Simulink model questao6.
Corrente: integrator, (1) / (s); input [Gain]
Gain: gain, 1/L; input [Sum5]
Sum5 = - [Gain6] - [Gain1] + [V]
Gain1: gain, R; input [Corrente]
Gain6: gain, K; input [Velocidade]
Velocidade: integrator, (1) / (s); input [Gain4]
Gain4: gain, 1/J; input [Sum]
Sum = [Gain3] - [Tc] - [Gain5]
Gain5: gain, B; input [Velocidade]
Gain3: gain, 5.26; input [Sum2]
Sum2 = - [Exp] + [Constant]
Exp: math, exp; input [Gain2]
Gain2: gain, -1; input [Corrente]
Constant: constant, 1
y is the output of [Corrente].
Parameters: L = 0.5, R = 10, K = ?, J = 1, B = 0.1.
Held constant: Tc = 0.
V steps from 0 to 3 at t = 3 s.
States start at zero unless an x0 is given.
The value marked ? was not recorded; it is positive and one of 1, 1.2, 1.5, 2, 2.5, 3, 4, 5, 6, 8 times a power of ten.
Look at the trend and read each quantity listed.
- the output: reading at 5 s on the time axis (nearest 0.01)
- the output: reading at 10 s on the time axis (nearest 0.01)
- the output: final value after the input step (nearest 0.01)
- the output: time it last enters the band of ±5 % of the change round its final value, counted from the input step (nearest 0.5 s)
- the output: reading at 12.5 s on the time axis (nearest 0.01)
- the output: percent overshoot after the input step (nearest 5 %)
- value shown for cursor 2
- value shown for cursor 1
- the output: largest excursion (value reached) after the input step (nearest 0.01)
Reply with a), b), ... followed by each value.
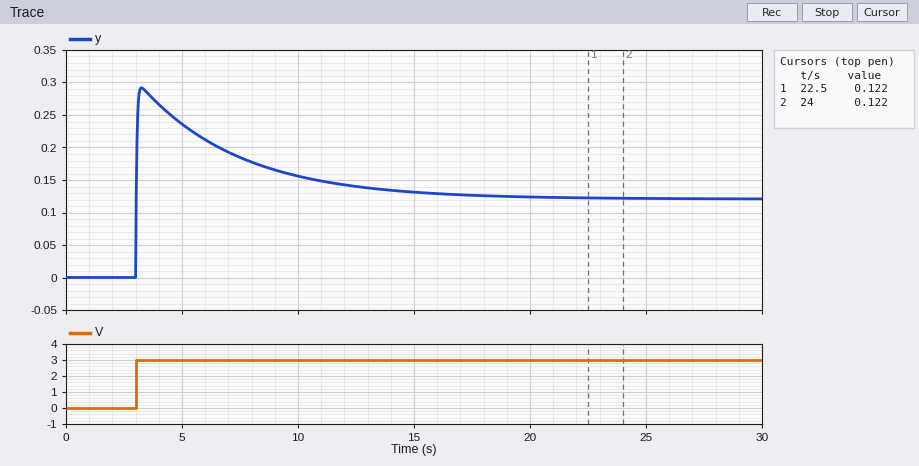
a) 0.24
b) 0.16
c) 0.12
d) 14.5 s
e) 0.14
f) 140 %
g) 0.122
h) 0.122
i) 0.29
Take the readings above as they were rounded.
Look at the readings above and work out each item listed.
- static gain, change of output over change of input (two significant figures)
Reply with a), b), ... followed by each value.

a) 0.040
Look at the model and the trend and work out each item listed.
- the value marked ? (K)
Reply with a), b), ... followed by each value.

a) 0.3
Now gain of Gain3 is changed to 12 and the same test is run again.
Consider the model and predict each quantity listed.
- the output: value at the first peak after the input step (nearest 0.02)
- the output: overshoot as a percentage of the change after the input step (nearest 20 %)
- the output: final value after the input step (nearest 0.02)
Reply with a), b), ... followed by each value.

a) 0.28
b) 320 %
c) 0.06
